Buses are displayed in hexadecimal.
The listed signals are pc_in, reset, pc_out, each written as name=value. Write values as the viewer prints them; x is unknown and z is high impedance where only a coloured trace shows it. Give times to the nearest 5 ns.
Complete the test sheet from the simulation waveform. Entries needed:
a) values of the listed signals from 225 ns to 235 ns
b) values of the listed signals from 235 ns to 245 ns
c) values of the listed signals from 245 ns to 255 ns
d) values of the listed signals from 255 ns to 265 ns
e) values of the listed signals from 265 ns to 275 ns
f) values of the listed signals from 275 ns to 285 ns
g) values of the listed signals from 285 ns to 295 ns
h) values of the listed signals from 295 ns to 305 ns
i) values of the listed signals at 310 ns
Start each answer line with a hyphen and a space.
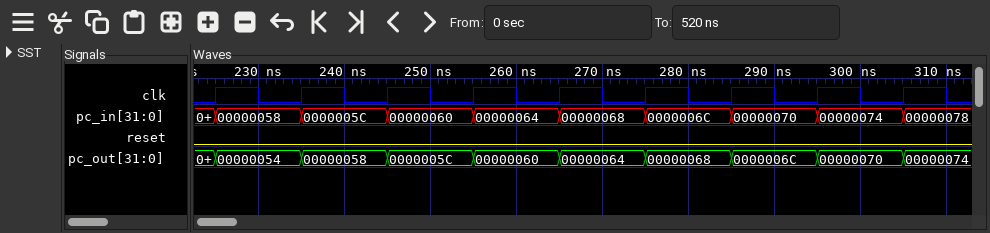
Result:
- pc_in=00000058, reset=0, pc_out=00000054
- pc_in=0000005C, reset=0, pc_out=00000058
- pc_in=00000060, reset=0, pc_out=0000005C
- pc_in=00000064, reset=0, pc_out=00000060
- pc_in=00000068, reset=0, pc_out=00000064
- pc_in=0000006C, reset=0, pc_out=00000068
- pc_in=00000070, reset=0, pc_out=0000006C
- pc_in=00000074, reset=0, pc_out=00000070
- pc_in=00000078, reset=0, pc_out=00000074
